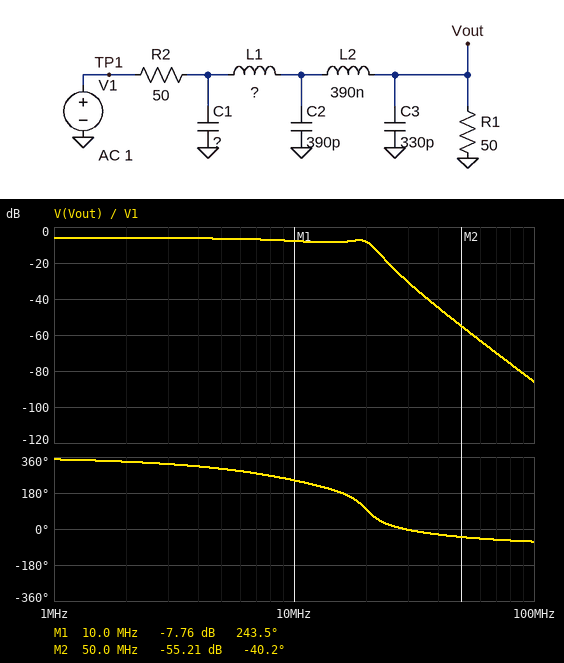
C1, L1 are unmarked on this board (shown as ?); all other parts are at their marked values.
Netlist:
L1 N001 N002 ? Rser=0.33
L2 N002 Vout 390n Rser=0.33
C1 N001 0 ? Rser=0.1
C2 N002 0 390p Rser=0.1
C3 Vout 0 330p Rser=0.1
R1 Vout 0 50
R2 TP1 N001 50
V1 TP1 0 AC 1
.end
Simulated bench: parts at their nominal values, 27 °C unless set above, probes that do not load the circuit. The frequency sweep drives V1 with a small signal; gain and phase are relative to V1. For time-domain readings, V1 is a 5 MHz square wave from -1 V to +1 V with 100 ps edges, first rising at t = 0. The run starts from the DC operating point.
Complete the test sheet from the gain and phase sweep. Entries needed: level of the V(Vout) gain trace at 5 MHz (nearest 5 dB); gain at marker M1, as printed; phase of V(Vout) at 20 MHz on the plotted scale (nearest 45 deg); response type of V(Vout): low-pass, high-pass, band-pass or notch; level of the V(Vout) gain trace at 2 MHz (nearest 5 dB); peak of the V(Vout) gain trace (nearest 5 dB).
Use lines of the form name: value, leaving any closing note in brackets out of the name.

level of the V(Vout) gain trace at 5 MHz: -5 dB
gain at marker M1, as printed: -7.76 dB
phase of V(Vout) at 20 MHz on the plotted scale: 90 deg
response type of V(Vout): low-pass, high-pass, band-pass or notch: low-pass
level of the V(Vout) gain trace at 2 MHz: -5 dB
peak of the V(Vout) gain trace: -5 dB
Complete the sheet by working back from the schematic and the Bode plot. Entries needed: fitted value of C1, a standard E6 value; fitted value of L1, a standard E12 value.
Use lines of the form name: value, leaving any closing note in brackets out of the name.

fitted value of C1, a standard E6 value: 100 pF
fitted value of L1, a standard E12 value: 820 nH
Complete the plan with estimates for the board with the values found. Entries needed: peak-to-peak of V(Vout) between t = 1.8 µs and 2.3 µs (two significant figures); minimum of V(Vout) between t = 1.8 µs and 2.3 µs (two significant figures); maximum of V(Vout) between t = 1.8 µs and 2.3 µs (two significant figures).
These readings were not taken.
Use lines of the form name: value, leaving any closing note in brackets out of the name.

peak-to-peak of V(Vout) between t = 1.8 µs and 2.3 µs: 1.1 V
minimum of V(Vout) between t = 1.8 µs and 2.3 µs: -540 mV
maximum of V(Vout) between t = 1.8 µs and 2.3 µs: 540 mV
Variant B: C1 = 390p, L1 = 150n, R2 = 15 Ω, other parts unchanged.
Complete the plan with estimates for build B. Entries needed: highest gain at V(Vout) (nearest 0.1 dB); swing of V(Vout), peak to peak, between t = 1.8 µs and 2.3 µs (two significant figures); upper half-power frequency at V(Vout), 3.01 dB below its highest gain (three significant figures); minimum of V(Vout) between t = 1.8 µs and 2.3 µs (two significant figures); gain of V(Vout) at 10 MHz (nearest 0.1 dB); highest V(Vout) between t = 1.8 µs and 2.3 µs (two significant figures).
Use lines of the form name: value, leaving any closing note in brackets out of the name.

highest gain at V(Vout): -1.1 dB
swing of V(Vout), peak to peak, between t = 1.8 µs and 2.3 µs: 2.1 V
upper half-power frequency at V(Vout), 3.01 dB below its highest gain: 19.3 MHz
minimum of V(Vout) between t = 1.8 µs and 2.3 µs: -1.0 V
gain of V(Vout) at 10 MHz: -1.2 dB
highest V(Vout) between t = 1.8 µs and 2.3 µs: 1.0 V
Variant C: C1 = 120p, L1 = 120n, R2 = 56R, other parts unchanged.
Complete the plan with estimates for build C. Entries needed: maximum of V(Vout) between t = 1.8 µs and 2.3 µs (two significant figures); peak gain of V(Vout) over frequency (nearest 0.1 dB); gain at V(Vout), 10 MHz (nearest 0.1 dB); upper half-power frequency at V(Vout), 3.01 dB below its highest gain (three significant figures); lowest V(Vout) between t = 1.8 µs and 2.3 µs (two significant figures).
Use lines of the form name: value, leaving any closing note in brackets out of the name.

maximum of V(Vout) between t = 1.8 µs and 2.3 µs: 490 mV
peak gain of V(Vout) over frequency: -6.6 dB
gain at V(Vout), 10 MHz: -8.2 dB
upper half-power frequency at V(Vout), 3.01 dB below its highest gain: 19.8 MHz
lowest V(Vout) between t = 1.8 µs and 2.3 µs: -490 mV
